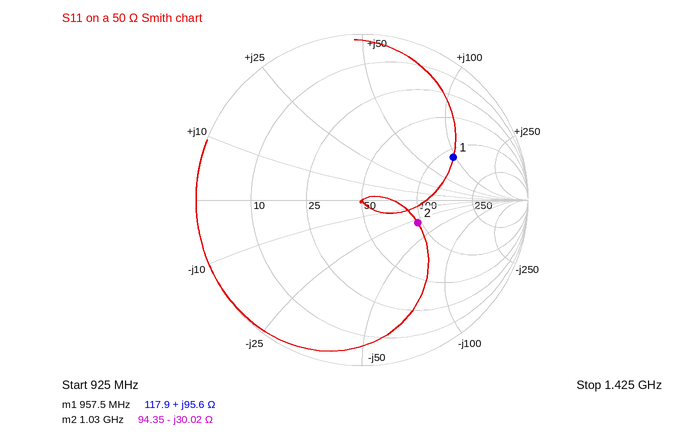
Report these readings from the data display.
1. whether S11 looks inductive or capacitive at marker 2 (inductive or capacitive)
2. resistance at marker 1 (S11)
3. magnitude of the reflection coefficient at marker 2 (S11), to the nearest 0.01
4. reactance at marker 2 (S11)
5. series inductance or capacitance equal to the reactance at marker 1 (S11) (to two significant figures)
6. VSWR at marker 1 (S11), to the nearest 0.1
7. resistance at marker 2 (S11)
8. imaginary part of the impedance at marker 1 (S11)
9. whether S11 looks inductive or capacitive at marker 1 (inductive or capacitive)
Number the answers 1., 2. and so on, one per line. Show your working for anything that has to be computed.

1. capacitive
2. 117.9 Ω
3. 0.36
4. -30.02 Ω
5. L = 95.6 Ω/(2π × 957.5 MHz) ≈ 16 nH
6. 4.1
7. 94.35 Ω
8. +95.6 Ω
9. inductive
